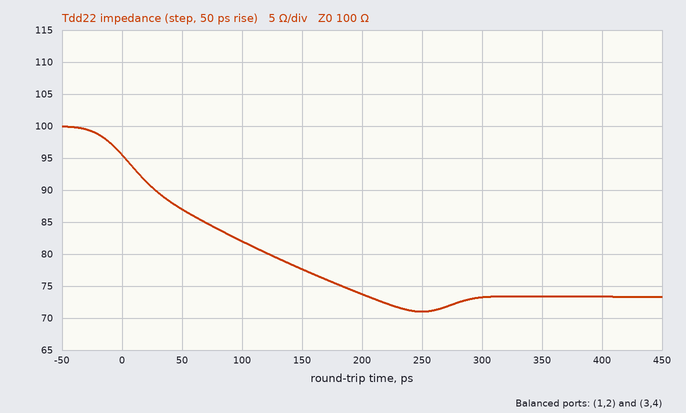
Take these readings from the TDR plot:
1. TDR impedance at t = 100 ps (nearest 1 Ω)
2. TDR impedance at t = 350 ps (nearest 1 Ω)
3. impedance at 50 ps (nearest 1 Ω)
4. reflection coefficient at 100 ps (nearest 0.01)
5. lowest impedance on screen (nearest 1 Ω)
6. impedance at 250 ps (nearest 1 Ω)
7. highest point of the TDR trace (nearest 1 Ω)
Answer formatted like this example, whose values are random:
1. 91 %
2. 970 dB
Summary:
1. 82 Ω
2. 73 Ω
3. 87 Ω
4. -0.10
5. 71 Ω
6. 71 Ω
7. 100 Ω
